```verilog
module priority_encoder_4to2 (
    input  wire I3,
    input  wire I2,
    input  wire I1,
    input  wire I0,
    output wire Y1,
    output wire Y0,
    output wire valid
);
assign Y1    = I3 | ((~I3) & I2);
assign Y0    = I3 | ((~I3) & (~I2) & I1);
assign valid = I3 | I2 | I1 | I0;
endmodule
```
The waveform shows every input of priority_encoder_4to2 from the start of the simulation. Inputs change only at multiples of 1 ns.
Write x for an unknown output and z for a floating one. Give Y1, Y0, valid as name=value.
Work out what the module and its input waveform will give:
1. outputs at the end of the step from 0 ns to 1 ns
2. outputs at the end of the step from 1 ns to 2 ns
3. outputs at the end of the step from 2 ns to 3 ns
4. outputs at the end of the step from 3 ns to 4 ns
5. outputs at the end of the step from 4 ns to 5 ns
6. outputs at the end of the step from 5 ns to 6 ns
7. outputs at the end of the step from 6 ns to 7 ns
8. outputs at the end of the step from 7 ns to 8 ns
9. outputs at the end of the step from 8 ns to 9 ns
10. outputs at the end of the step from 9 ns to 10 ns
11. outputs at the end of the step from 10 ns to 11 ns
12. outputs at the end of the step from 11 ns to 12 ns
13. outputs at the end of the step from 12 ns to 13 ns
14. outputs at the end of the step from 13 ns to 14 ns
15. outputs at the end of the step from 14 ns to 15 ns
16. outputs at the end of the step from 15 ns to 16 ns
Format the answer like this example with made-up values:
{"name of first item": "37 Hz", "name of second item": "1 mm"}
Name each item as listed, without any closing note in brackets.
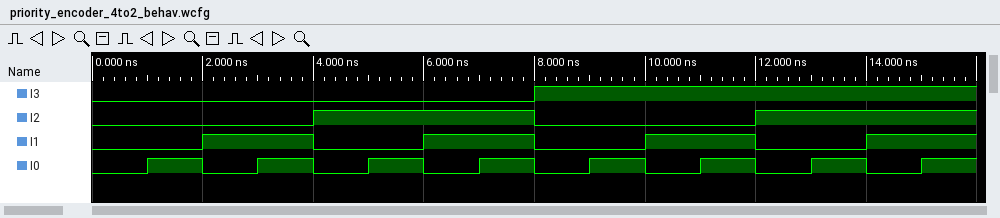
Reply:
{"outputs at the end of the step from 0 ns to 1 ns": "Y1=0, Y0=0, valid=0", "outputs at the end of the step from 1 ns to 2 ns": "Y1=0, Y0=0, valid=1", "outputs at the end of the step from 2 ns to 3 ns": "Y1=0, Y0=1, valid=1", "outputs at the end of the step from 3 ns to 4 ns": "Y1=0, Y0=1, valid=1", "outputs at the end of the step from 4 ns to 5 ns": "Y1=1, Y0=0, valid=1", "outputs at the end of the step from 5 ns to 6 ns": "Y1=1, Y0=0, valid=1", "outputs at the end of the step from 6 ns to 7 ns": "Y1=1, Y0=0, valid=1", "outputs at the end of the step from 7 ns to 8 ns": "Y1=1, Y0=0, valid=1", "outputs at the end of the step from 8 ns to 9 ns": "Y1=1, Y0=1, valid=1", "outputs at the end of the step from 9 ns to 10 ns": "Y1=1, Y0=1, valid=1", "outputs at the end of the step from 10 ns to 11 ns": "Y1=1, Y0=1, valid=1", "outputs at the end of the step from 11 ns to 12 ns": "Y1=1, Y0=1, valid=1", "outputs at the end of the step from 12 ns to 13 ns": "Y1=1, Y0=1, valid=1", "outputs at the end of the step from 13 ns to 14 ns": "Y1=1, Y0=1, valid=1", "outputs at the end of the step from 14 ns to 15 ns": "Y1=1, Y0=1, valid=1", "outputs at the end of the step from 15 ns to 16 ns": "Y1=1, Y0=1, valid=1"}
